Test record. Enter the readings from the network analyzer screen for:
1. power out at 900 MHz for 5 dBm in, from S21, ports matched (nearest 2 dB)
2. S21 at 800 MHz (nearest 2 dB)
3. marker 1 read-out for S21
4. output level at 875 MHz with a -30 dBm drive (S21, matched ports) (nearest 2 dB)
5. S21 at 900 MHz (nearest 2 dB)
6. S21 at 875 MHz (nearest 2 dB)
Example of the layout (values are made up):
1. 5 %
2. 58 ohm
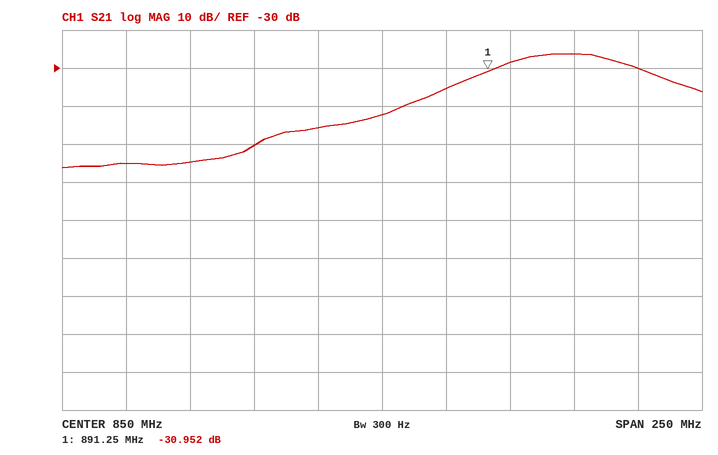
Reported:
1. -24 dBm
2. -50 dB
3. -30.952 dB
4. -66 dBm
5. -28 dB
6. -36 dB
